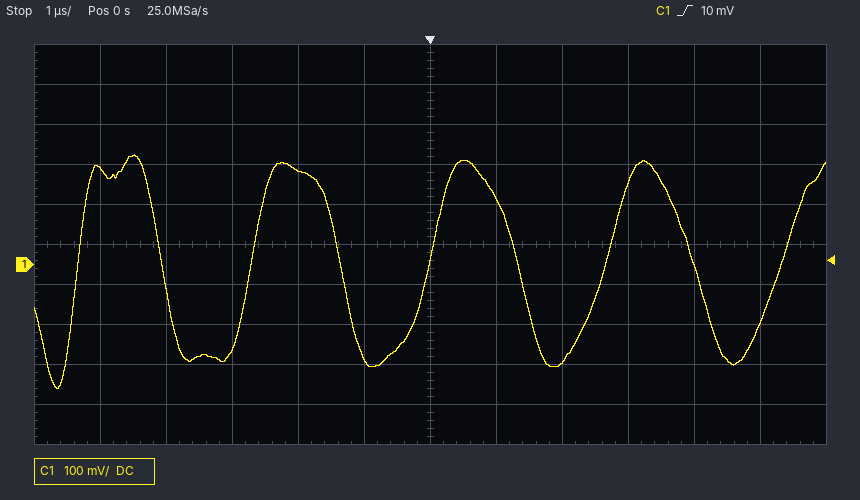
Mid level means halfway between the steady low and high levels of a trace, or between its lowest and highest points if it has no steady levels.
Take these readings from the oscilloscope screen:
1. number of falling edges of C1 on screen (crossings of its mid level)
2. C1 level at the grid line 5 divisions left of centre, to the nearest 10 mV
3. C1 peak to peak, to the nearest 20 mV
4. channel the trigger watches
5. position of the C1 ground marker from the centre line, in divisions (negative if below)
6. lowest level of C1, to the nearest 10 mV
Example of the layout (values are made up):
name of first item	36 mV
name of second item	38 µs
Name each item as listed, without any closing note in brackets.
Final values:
number of falling edges of C1 on screen	4
C1 level at the grid line 5 divisions left of centre, to the nearest 10 mV	240 mV
C1 peak to peak, to the nearest 20 mV	580 mV
channel the trigger watches	C1
position of the C1 ground marker from the centre line, in divisions	-0.5 div
lowest level of C1, to the nearest 10 mV	-310 mV
